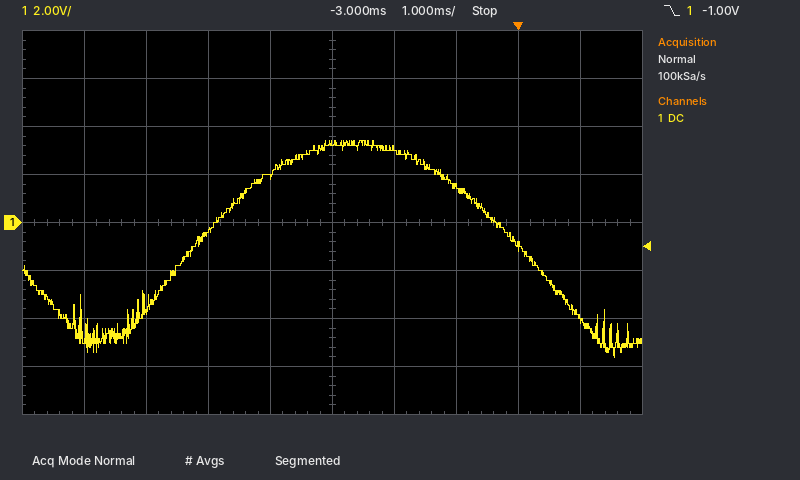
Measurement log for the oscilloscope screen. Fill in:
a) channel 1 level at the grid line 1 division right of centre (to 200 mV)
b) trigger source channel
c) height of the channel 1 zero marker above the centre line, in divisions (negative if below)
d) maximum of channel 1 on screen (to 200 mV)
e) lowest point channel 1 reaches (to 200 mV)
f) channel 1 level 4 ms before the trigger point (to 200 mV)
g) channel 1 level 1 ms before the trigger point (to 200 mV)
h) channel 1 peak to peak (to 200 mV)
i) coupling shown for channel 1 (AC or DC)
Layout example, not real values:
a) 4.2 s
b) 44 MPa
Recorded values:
a) 3.0 V
b) channel 1
c) 0.0 div
d) 3.4 V
e) -5.6 V
f) 2.0 V
g) 1.4 V
h) 9.0 V
i) DC
